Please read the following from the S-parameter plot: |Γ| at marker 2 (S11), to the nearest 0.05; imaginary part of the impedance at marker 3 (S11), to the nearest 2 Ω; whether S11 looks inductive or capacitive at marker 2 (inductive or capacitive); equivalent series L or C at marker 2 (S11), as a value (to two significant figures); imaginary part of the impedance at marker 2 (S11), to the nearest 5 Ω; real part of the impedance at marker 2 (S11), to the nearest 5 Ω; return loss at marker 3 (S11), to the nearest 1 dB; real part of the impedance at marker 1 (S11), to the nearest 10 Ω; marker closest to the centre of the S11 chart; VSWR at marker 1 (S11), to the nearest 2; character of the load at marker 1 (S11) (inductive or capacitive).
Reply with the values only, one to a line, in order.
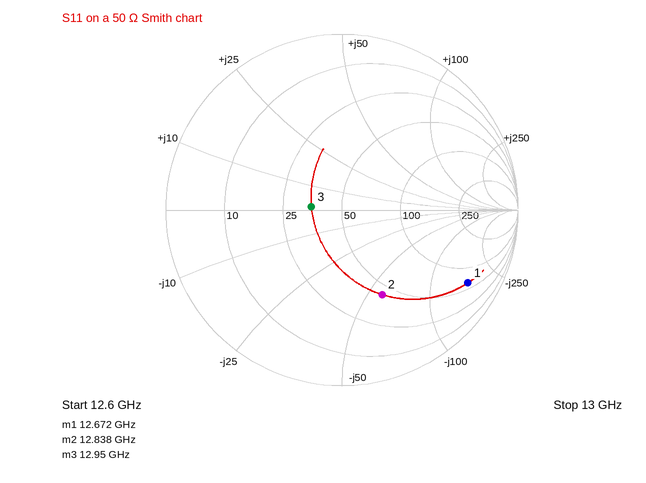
0.55
+2 Ω
capacitive
210 fF
-60 Ω
45 Ω
15 dB
60 Ω
marker 3
10
capacitive
